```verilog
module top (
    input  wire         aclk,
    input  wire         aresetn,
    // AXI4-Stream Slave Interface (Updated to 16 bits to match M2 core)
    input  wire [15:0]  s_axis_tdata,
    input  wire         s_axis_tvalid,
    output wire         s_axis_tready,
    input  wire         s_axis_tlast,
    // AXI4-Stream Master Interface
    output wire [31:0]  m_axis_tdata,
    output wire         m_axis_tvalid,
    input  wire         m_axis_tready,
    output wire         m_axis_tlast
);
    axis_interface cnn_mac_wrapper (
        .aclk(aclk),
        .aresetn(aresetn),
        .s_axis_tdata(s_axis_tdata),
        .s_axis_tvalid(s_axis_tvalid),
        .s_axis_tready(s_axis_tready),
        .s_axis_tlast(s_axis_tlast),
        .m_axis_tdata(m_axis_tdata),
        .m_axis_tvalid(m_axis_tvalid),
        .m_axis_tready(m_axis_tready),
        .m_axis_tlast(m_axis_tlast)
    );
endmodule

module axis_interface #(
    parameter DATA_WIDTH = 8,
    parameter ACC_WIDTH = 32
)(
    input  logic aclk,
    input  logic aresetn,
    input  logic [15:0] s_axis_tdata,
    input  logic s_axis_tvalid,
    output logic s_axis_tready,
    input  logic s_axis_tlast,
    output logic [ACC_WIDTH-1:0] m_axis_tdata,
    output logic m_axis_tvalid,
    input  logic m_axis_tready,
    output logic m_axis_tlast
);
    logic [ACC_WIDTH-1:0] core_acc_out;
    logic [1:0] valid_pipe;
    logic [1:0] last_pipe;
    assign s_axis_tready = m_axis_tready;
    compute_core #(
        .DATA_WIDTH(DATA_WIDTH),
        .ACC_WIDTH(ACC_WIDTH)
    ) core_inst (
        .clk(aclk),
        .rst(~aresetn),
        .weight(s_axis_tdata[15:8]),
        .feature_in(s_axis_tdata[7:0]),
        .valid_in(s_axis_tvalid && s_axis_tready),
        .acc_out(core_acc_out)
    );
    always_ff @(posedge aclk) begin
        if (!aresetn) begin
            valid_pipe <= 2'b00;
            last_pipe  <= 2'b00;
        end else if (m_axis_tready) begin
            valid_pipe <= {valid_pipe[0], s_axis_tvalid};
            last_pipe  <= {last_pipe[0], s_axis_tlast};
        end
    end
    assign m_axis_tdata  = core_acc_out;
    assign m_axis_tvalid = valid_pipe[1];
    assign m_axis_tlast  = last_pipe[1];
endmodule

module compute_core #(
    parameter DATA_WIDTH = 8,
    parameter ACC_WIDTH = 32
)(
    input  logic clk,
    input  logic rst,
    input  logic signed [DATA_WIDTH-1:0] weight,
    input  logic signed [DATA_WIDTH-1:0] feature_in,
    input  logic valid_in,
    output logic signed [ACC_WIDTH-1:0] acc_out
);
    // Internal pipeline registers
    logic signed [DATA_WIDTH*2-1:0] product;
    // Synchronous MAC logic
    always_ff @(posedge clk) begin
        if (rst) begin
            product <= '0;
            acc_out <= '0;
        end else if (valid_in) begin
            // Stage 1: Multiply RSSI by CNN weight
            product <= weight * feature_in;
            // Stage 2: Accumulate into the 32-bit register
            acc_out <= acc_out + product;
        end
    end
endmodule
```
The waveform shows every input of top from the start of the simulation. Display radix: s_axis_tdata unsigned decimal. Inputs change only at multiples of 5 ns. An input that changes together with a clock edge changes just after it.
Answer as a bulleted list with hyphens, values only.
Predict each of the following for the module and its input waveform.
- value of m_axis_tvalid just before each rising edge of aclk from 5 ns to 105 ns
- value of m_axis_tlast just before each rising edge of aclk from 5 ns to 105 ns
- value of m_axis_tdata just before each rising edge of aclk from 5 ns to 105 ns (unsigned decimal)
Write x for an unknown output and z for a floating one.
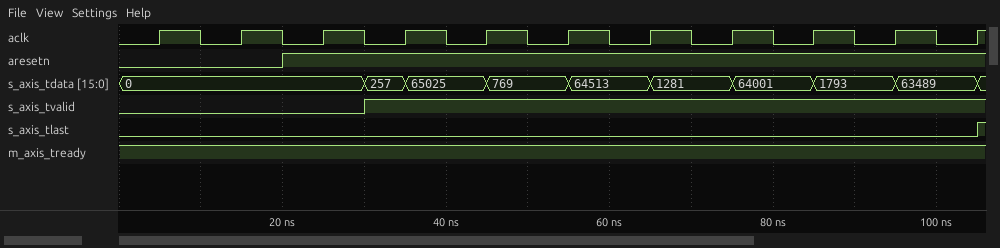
- x 0 0 0 0 1 1 1 1 1 1
- x 0 0 0 0 0 0 0 0 0 0
- x, 0, 0, 0, 0, 1, 4294967295, 2, 4294967294, 3, 4294967293
